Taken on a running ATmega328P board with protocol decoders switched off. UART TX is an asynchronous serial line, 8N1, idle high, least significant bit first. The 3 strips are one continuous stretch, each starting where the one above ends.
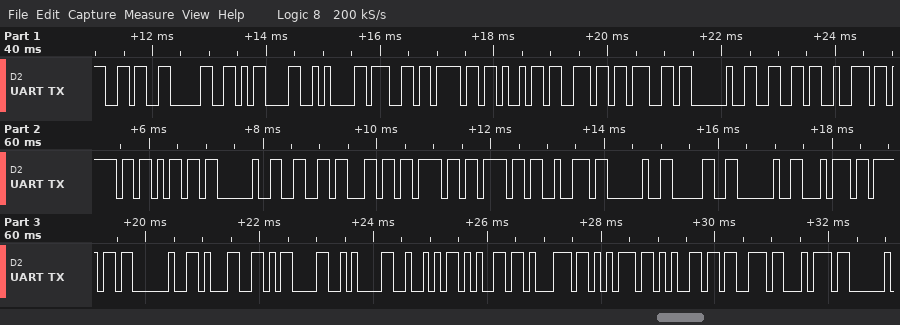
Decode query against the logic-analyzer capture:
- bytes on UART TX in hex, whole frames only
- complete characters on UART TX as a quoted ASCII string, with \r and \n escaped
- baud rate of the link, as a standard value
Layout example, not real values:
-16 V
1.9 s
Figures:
0x36 0x30 0x0D 0x0A 0x67 0x6F 0x69 0x6E 0x67 0x20 0x66 0x72 0x6F 0x6D 0x20 0x66 0x6C 0x6F 0x6F 0x72 0x20 0x30 0x20 0x74 0x6F 0x20 0x31 0x0D 0x0A 0x52 0x65 0x71 0x75 0x65 0x73 0x74
"60\r\ngoing from floor 0 to 1\r\nRequest"
9600 baud
